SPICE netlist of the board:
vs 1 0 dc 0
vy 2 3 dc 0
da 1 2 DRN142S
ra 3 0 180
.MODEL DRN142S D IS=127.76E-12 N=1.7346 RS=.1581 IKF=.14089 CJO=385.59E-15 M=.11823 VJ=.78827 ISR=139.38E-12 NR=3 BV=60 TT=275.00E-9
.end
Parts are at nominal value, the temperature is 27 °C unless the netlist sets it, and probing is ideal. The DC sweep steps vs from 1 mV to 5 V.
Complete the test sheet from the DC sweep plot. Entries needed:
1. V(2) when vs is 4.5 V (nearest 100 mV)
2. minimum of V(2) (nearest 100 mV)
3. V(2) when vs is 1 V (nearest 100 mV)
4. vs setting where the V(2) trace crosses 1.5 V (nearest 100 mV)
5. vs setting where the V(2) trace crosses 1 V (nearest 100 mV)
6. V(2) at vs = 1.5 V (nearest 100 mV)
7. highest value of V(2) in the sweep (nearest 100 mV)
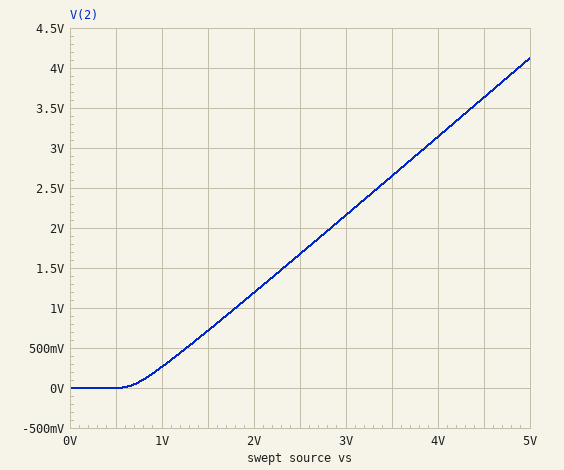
3.6 V
0 V
300 mV
2.3 V
1.8 V
700 mV
4.1 V
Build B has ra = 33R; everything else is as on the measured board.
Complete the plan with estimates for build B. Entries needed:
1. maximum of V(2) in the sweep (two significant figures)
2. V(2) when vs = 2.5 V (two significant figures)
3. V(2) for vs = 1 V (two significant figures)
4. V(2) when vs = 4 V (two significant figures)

4.0 V
1.6 V
200 mV
3.0 V
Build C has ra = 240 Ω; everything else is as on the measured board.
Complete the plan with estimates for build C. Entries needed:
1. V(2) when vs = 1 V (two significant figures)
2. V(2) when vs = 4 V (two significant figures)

280 mV
3.2 V
